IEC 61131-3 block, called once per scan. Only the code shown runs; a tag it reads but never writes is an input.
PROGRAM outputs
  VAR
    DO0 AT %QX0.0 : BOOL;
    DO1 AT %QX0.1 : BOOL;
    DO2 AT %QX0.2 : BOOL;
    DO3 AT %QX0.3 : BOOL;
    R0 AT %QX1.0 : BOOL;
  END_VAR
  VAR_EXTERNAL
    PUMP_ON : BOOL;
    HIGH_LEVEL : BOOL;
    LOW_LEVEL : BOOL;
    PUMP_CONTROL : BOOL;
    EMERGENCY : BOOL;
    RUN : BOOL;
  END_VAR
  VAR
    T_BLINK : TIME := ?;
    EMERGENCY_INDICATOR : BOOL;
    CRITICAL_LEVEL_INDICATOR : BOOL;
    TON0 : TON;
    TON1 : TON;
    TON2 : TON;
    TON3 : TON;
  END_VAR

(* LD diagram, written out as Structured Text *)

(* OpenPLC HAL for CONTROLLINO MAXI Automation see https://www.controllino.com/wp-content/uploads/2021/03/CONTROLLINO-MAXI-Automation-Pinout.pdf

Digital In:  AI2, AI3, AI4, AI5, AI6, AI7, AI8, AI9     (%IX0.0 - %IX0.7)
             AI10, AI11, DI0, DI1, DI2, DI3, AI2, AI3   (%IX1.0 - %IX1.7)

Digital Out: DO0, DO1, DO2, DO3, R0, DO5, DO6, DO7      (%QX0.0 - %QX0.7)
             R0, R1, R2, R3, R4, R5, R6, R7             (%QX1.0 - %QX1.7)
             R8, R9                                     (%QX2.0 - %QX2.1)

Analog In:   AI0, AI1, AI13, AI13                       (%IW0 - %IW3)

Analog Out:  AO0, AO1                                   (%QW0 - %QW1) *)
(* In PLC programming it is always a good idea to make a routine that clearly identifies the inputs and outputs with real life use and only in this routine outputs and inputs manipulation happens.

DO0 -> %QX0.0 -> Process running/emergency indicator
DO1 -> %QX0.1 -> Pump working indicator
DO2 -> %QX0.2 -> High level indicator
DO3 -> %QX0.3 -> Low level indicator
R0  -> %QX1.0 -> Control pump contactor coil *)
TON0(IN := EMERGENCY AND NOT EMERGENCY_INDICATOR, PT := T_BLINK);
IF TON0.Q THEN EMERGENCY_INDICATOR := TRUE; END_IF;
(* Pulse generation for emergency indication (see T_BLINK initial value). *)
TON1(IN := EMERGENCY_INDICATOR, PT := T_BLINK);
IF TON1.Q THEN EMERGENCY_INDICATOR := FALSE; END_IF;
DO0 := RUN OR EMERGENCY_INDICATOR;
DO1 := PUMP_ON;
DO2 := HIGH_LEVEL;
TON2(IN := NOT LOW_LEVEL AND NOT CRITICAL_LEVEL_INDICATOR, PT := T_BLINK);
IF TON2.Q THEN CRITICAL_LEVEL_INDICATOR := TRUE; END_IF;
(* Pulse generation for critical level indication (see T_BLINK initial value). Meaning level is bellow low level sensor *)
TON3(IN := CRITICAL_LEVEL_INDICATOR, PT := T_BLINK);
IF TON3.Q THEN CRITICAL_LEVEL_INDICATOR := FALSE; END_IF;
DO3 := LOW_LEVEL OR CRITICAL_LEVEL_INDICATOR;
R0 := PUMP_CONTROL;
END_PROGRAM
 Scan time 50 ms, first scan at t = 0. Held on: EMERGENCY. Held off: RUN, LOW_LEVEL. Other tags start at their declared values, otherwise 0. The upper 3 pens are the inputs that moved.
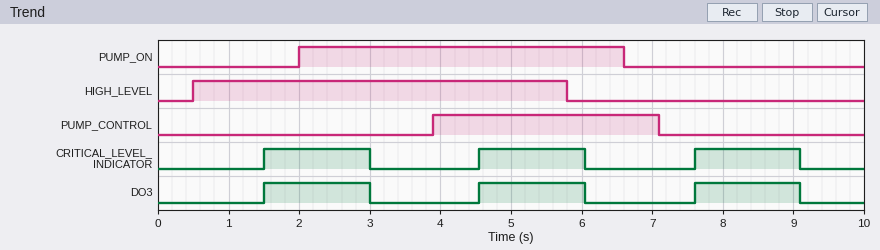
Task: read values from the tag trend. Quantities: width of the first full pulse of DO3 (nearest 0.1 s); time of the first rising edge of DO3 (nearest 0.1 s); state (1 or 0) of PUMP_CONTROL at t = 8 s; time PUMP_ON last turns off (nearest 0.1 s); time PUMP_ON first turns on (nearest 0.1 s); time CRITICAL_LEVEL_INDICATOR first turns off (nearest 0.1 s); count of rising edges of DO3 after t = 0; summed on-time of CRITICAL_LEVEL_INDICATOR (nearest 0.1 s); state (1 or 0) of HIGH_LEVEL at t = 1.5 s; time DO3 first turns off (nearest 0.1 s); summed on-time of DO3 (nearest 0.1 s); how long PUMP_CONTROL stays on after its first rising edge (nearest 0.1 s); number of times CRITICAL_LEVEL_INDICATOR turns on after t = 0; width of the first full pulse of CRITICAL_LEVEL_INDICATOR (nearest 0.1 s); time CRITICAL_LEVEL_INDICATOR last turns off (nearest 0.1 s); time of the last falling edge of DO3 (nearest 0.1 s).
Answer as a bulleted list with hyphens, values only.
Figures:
- 1.5 s
- 1.5 s
- 0
- 6.6 s
- 2.0 s
- 3.0 s
- 3
- 4.5 s
- 1
- 3.0 s
- 4.5 s
- 3.2 s
- 3
- 1.5 s
- 9.1 s
- 9.1 s
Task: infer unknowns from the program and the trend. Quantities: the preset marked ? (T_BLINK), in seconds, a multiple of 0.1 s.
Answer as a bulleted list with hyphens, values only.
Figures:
- 1.5 s
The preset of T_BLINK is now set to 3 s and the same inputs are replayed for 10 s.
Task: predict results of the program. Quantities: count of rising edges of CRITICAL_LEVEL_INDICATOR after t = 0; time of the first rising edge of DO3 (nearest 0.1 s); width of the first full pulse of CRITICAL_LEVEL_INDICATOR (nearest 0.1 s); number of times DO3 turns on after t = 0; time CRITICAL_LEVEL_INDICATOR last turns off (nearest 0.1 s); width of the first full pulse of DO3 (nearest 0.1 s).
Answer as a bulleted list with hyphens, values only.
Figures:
- 2
- 3.0 s
- 3.0 s
- 2
- 6.0 s
- 3.0 s
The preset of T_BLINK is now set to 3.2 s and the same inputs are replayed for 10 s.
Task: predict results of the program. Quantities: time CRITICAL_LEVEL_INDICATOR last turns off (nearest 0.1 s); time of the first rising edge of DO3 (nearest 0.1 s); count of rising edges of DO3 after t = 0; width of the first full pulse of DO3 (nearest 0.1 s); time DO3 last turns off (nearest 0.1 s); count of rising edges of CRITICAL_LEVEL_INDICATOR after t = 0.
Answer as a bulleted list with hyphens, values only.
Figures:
- 6.4 s
- 3.2 s
- 2
- 3.2 s
- 6.4 s
- 2
